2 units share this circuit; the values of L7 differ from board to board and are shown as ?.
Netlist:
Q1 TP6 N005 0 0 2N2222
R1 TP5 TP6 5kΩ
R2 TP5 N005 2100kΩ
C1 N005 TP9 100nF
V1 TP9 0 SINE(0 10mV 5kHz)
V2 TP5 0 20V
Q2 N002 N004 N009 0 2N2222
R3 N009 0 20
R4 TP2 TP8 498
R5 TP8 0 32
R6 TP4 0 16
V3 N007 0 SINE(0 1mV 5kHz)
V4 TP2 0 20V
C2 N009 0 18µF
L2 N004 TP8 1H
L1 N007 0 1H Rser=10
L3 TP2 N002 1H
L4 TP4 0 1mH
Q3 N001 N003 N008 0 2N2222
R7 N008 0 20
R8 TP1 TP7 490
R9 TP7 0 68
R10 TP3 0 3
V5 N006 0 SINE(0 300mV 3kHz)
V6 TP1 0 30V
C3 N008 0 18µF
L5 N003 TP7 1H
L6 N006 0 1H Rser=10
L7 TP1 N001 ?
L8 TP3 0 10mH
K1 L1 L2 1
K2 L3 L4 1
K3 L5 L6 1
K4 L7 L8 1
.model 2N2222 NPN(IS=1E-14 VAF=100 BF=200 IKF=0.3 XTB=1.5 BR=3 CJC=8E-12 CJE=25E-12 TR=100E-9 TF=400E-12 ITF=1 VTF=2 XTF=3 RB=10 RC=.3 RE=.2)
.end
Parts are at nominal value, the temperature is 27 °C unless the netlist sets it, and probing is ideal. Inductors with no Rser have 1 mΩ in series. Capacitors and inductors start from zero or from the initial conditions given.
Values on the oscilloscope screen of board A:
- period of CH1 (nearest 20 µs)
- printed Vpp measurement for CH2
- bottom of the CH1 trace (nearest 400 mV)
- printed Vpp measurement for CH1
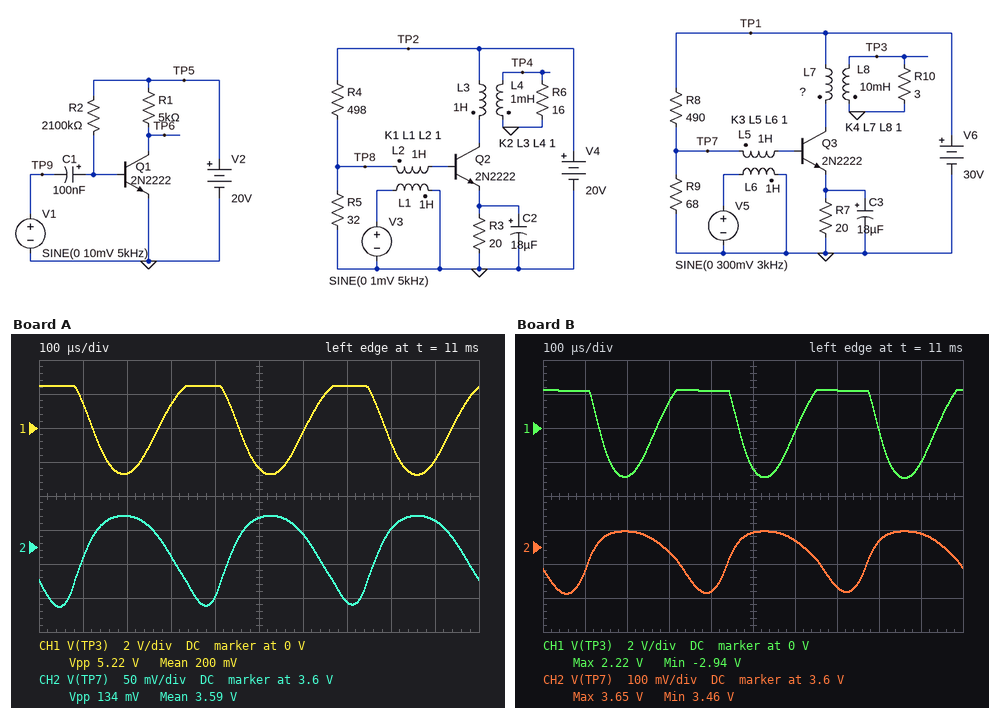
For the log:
340 µs
134 mV
-2.8 V
5.22 V
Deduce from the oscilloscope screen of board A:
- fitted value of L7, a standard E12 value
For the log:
1.2 H
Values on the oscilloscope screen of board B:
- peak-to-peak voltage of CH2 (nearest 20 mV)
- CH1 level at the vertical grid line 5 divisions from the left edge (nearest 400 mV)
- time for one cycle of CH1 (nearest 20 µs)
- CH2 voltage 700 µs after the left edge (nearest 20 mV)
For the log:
180 mV
-2.4 V
340 µs
3.48 V
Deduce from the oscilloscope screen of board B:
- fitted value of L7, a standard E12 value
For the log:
1.5 H
